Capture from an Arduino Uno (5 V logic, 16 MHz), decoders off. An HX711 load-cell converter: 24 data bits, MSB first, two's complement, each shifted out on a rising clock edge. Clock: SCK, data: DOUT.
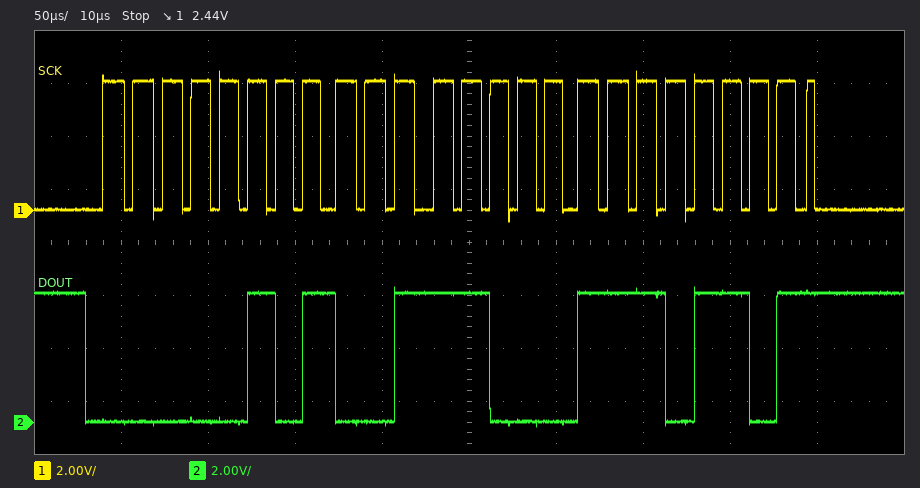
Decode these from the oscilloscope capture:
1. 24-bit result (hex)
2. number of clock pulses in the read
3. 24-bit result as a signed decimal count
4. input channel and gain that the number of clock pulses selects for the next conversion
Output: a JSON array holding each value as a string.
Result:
["0x0538ED", "25", "342253", "channel A, gain 128"]
